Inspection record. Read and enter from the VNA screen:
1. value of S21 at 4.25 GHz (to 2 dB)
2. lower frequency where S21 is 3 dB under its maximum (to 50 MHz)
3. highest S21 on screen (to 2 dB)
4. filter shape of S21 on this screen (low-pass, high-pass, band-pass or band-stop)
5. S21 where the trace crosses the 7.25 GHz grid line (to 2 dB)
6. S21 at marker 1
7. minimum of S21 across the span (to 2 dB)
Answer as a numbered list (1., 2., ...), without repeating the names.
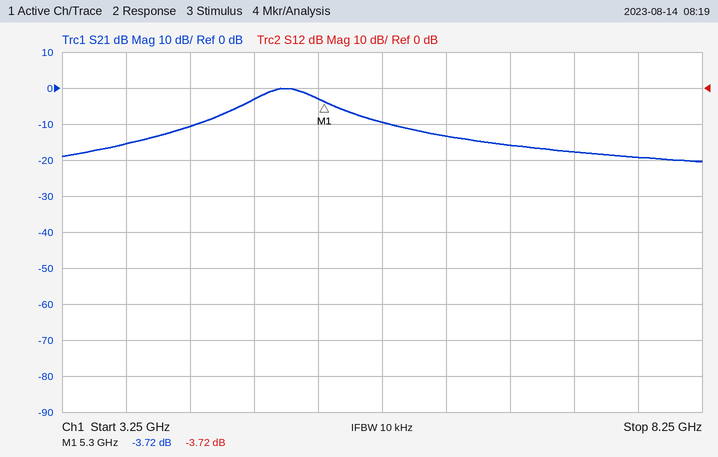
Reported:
1. -10 dB
2. 4.75 GHz
3. 0 dB
4. band-pass
5. -18 dB
6. -3.72 dB
7. -20 dB
